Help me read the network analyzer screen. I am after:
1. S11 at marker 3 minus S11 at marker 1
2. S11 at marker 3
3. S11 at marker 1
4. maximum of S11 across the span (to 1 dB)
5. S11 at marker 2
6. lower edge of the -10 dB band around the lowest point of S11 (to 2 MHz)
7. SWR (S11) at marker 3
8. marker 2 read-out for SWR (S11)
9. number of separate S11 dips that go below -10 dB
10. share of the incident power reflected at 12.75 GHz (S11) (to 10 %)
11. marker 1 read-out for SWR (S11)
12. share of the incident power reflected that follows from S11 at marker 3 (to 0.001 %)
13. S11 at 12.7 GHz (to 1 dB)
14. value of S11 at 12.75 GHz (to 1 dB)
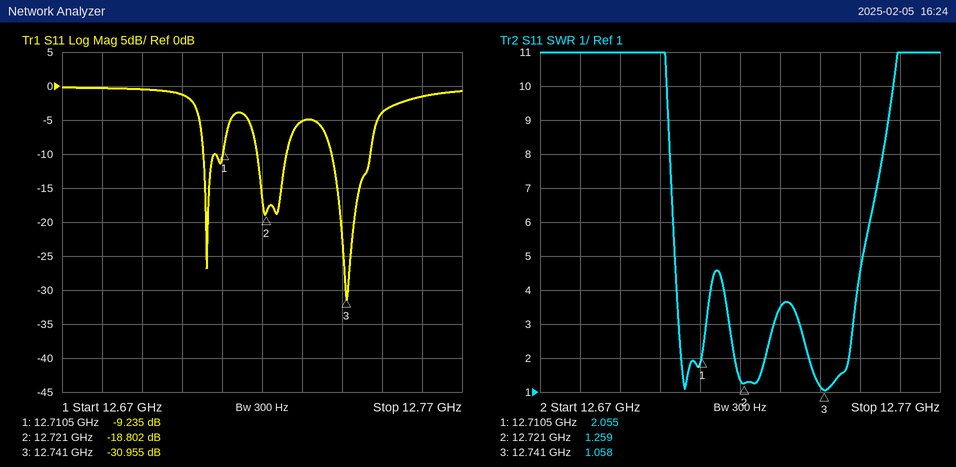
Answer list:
-21.720 dB
-30.955 dB
-9.235 dB
0 dB
-18.802 dB
12.738 GHz
1.058
1.259
3
40 %
2.055
0.080 %
-1 dB
-4 dB
